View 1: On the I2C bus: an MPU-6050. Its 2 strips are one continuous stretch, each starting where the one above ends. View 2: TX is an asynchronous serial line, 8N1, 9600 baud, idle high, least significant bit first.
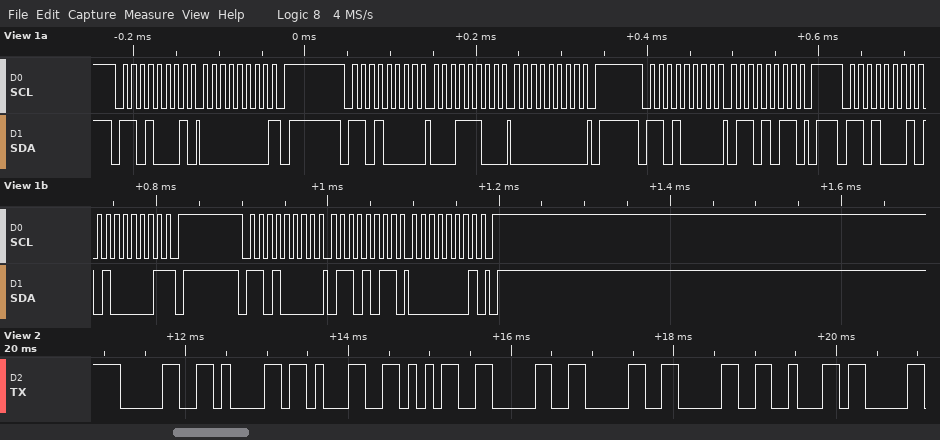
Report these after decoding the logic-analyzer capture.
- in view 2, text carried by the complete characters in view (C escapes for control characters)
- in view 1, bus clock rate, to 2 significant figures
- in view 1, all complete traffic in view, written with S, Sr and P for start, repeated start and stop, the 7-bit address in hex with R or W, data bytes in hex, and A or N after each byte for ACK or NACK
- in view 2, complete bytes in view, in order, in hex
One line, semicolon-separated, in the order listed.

"0a15000b"; 100 kHz; S 68R A 00 N P S 68W A 1C A 00 A P S 68W A 6B A P S 68R A 41 N P S 68W A 6B A 01 A P; 30 61 31 35 30 30 30 62
